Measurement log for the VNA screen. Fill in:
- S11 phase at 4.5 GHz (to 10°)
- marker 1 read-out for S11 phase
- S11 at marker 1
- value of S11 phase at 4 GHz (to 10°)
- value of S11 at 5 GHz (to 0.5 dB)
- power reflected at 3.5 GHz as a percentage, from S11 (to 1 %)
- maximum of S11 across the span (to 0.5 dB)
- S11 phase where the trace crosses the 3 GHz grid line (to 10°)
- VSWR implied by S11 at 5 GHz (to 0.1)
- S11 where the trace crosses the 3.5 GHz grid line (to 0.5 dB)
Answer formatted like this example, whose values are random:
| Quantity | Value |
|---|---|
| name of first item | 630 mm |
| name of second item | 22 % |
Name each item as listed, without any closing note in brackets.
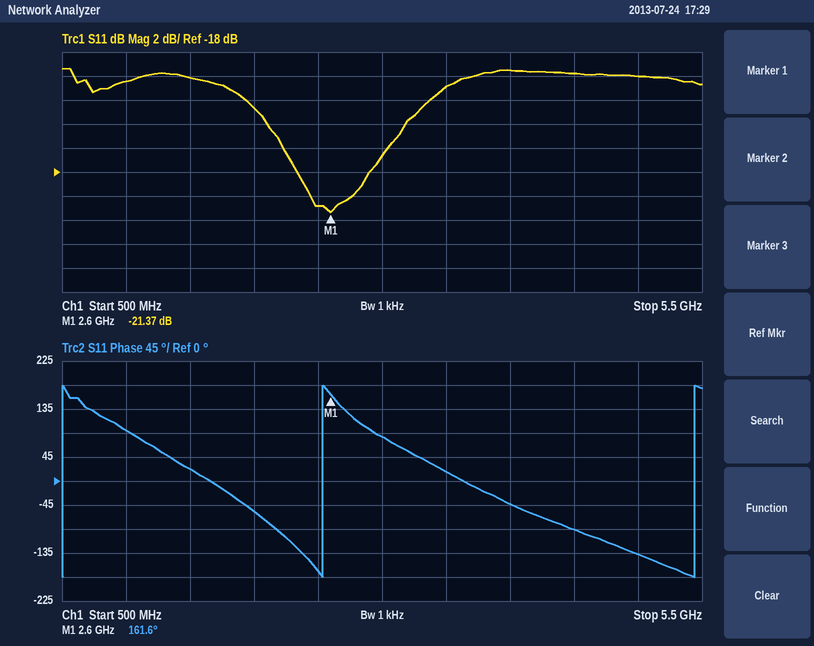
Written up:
| Quantity | Value |
|---|---|
| S11 phase at 4.5 GHz | -90° |
| marker 1 read-out for S11 phase | 161.6° |
| S11 at marker 1 | -21.37 dB |
| value of S11 phase at 4 GHz | -40° |
| value of S11 at 5 GHz | -10.0 dB |
| power reflected at 3.5 GHz as a percentage, from S11 | 8 % |
| maximum of S11 across the span | -9.5 dB |
| S11 phase where the trace crosses the 3 GHz grid line | 80° |
| VSWR implied by S11 at 5 GHz | 1.9 |
| S11 where the trace crosses the 3.5 GHz grid line | -11.0 dB |
